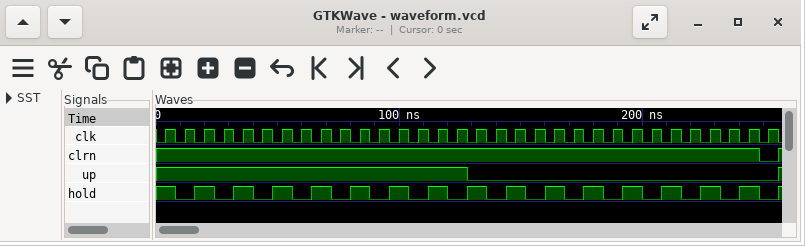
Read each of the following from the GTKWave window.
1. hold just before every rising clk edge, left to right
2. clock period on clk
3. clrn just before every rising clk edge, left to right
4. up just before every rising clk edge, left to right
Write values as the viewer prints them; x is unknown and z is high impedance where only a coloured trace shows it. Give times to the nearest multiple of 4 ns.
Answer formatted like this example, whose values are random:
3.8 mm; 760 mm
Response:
1 0 1 0 1 0 1 0 1 0 1 0 1 0 1 0 1 0 1 0 1 0 1 0 1 0 1 0 1 0 1 0; 8 ns; 1 1 1 1 1 1 1 1 1 1 1 1 1 1 1 1 1 1 1 1 1 1 1 1 1 1 1 1 1 1 1 0; 1 1 1 1 1 1 1 1 1 1 1 1 1 1 1 1 0 0 0 0 0 0 0 0 0 0 0 0 0 0 0 0
